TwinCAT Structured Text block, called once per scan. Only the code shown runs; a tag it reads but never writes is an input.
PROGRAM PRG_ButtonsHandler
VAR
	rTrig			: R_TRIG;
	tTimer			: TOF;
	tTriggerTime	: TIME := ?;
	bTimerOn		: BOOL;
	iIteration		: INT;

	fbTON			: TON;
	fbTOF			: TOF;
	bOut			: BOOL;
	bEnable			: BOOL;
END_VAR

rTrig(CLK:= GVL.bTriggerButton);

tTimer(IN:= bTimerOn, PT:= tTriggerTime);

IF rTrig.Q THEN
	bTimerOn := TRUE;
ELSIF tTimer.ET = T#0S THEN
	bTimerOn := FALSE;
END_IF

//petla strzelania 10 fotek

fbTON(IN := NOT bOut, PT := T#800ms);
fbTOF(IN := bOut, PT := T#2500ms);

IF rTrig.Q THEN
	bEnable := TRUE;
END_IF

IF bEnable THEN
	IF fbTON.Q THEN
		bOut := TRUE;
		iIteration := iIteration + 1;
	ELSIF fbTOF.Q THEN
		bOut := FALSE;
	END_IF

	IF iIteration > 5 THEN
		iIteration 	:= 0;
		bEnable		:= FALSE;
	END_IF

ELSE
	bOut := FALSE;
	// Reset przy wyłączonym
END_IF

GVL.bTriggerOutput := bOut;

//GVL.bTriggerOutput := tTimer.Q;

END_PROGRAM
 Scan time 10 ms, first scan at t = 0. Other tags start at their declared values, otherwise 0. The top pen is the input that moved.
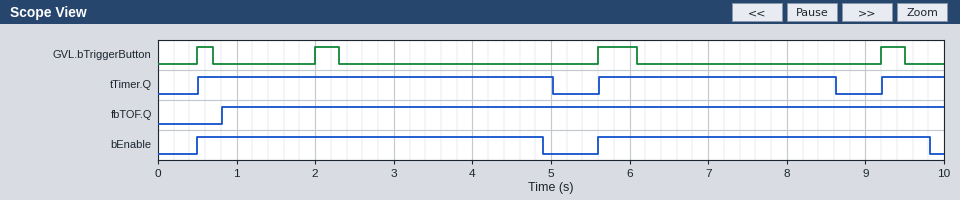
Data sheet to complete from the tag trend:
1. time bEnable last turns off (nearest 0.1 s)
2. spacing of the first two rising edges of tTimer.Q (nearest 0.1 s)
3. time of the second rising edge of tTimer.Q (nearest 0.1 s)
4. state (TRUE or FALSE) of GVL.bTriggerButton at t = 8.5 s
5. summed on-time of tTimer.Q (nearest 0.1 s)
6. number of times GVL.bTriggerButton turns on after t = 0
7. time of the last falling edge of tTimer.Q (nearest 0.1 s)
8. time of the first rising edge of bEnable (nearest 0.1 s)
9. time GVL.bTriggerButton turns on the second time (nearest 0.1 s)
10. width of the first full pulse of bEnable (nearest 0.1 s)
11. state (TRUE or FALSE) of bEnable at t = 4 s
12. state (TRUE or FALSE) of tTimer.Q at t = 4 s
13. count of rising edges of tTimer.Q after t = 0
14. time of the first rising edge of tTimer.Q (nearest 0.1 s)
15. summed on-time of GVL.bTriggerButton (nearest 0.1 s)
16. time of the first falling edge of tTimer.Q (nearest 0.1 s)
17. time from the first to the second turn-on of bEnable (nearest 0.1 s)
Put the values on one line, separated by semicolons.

9.8 s; 5.1 s; 5.6 s; FALSE; 8.3 s; 4; 8.6 s; 0.5 s; 2.0 s; 4.4 s; TRUE; TRUE; 3; 0.5 s; 1.3 s; 5.0 s; 5.1 s
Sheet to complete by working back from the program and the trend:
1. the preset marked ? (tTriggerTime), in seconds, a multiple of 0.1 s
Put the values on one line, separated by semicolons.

3.0 s
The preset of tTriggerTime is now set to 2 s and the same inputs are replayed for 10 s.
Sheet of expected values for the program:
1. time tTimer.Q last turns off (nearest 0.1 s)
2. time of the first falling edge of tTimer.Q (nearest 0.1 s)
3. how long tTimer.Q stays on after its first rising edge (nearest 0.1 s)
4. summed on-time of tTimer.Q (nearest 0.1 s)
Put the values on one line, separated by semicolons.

7.6 s; 4.0 s; 3.5 s; 6.3 s
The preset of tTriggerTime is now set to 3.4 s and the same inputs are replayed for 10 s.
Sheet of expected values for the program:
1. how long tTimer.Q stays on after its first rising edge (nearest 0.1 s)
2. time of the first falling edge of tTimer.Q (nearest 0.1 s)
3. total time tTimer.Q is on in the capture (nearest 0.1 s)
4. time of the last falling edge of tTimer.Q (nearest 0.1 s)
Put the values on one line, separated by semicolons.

4.9 s; 5.4 s; 9.1 s; 9.0 s
